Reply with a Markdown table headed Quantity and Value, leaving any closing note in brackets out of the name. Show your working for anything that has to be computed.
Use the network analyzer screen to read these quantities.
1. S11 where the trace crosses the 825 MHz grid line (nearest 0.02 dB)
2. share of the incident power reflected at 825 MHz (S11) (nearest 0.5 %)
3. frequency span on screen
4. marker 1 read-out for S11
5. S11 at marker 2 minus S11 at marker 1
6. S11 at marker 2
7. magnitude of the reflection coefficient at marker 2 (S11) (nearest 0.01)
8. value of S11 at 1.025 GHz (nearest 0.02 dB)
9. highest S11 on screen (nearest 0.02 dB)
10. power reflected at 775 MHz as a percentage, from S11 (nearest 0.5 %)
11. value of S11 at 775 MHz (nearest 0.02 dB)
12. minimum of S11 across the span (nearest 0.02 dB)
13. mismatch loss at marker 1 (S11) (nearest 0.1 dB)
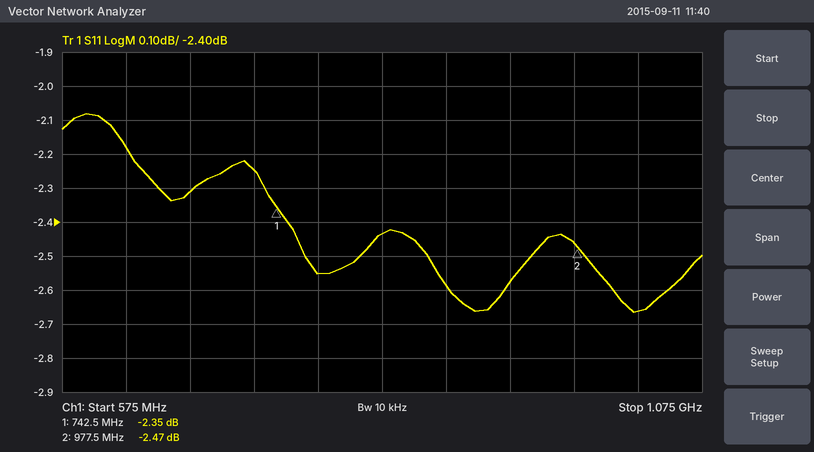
| Quantity | Value |
|---|---|
| S11 where the trace crosses the 825 MHz grid line | -2.44 dB |
| share of the incident power reflected at 825 MHz (S11) | 10^(-2.44/10) ≈ 57.0 % |
| frequency span on screen | 500 MHz |
| marker 1 read-out for S11 | -2.35 dB |
| S11 at marker 2 minus S11 at marker 1 | -2.47 − (-2.35) = -0.12 dB |
| S11 at marker 2 | -2.47 dB |
| magnitude of the reflection coefficient at marker 2 (S11) | 10^(-2.47/20) ≈ 0.75 |
| value of S11 at 1.025 GHz | -2.66 dB |
| highest S11 on screen | -2.08 dB |
| power reflected at 775 MHz as a percentage, from S11 | 10^(-2.56/10) ≈ 55.5 % |
| value of S11 at 775 MHz | -2.56 dB |
| minimum of S11 across the span | -2.66 dB |
| mismatch loss at marker 1 (S11) | −10 log10(1 − 10^(-2.35/10)) ≈ 3.8 dB |
